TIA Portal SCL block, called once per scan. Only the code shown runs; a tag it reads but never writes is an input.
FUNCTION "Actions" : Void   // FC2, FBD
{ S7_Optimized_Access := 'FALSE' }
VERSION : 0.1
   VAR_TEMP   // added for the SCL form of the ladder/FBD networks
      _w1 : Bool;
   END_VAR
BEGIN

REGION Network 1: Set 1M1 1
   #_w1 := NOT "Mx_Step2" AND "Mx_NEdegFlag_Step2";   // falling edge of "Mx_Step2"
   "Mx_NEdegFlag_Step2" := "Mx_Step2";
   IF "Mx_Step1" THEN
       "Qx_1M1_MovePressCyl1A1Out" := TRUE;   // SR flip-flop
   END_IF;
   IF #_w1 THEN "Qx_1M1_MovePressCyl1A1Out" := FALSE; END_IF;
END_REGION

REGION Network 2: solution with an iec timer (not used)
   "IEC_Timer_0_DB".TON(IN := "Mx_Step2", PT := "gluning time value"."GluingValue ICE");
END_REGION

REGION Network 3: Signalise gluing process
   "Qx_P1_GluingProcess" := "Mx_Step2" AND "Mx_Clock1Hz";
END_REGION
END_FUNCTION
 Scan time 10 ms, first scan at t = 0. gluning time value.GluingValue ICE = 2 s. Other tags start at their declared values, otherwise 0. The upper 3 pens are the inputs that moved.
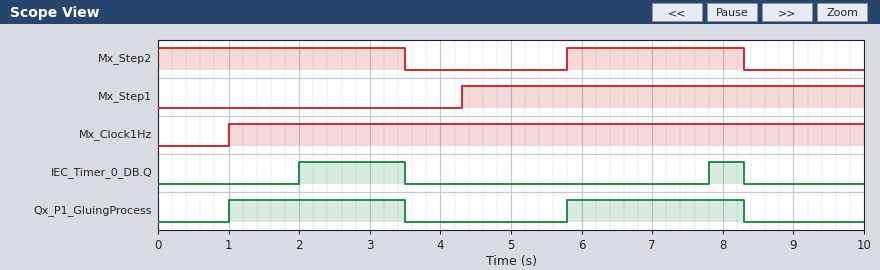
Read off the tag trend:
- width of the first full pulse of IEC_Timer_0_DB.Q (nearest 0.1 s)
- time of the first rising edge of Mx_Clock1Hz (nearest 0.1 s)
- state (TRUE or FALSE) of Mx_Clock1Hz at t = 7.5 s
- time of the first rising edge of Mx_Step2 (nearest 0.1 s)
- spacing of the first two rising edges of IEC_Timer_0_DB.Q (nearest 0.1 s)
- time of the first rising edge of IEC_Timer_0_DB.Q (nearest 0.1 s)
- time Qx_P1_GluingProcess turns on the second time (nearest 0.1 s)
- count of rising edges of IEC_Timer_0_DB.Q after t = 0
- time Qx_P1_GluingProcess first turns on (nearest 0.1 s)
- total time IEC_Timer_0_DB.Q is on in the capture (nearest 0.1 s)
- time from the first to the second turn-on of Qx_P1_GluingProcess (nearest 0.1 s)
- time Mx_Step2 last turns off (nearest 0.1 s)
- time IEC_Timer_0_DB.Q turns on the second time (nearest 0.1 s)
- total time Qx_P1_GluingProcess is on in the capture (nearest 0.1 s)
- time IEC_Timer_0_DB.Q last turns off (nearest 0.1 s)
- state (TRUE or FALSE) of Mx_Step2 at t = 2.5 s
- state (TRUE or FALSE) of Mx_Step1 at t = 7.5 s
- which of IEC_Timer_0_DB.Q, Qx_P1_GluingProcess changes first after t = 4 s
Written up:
1.5 s
1.0 s
TRUE
5.8 s
5.8 s
2.0 s
5.8 s
2
1.0 s
2.0 s
4.8 s
8.3 s
7.8 s
5.0 s
8.3 s
TRUE
TRUE
Qx_P1_GluingProcess
